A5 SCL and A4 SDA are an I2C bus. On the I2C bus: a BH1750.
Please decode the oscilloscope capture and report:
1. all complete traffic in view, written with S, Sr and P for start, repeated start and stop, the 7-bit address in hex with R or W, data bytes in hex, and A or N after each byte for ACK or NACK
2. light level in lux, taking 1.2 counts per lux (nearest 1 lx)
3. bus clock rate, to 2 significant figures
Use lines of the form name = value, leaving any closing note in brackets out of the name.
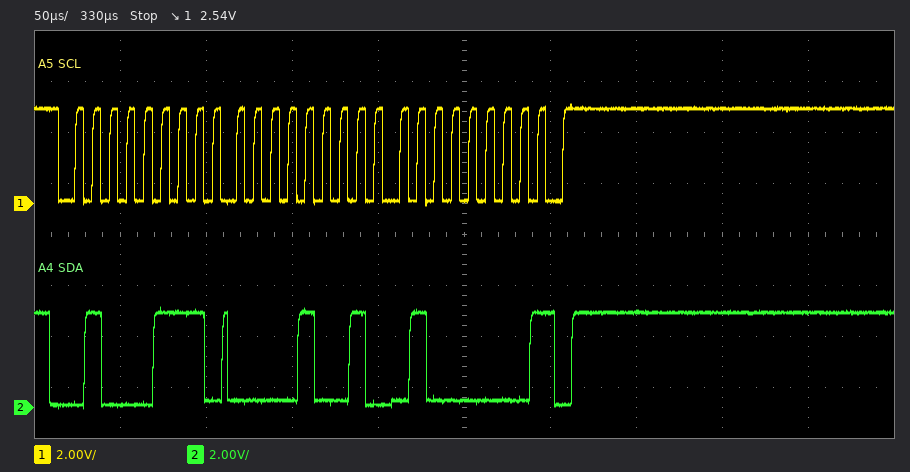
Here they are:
all complete traffic in view, written with S, Sr and P for start, repeated start and stop, the 7-bit address in hex with R or W, data bytes in hex, and A or N after each byte for ACK or NACK = S 23R A 09 A 40 N P
light level in lux, taking 1.2 counts per lux = 1973 lx
bus clock rate, to 2 significant figures = 100 kHz
